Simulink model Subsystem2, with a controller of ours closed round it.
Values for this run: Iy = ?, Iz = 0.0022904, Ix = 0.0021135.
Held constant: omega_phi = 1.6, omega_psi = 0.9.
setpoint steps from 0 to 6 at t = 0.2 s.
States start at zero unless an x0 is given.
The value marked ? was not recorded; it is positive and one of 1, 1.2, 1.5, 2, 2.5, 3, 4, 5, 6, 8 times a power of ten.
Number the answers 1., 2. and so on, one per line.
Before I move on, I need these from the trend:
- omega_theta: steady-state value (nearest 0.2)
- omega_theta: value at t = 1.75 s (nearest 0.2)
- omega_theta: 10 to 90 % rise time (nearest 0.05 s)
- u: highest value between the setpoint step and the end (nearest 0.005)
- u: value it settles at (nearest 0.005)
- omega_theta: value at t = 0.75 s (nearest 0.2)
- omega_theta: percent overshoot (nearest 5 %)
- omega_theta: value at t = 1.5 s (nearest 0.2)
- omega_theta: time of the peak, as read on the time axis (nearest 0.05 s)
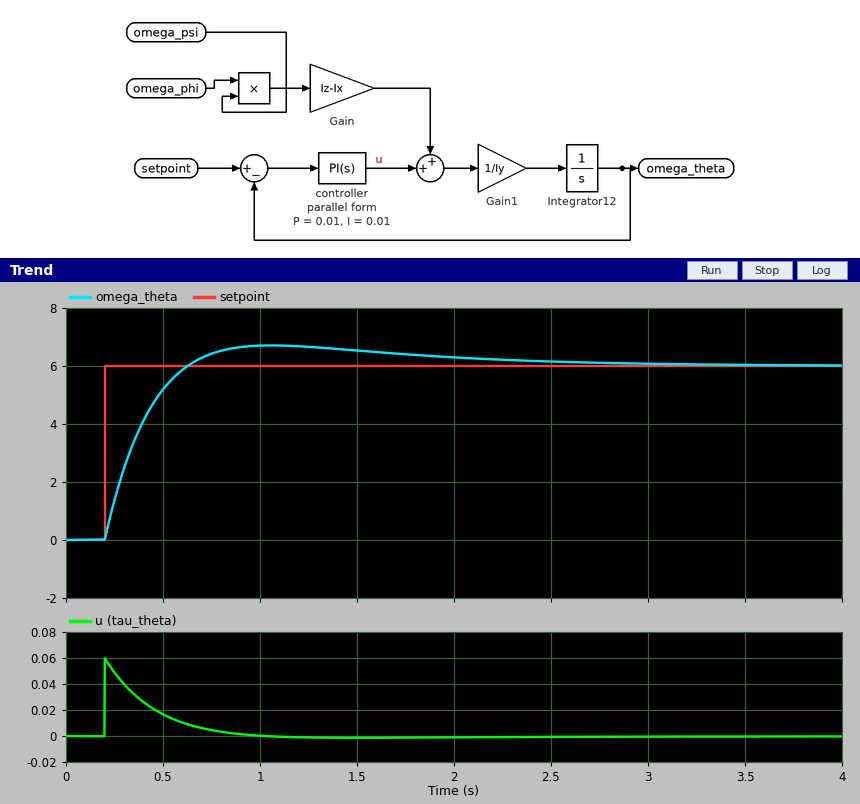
1. 6.0
2. 6.4
3. 0.30 s
4. 0.060
5. 0.000
6. 6.4
7. 10 %
8. 6.6
9. 1.05 s
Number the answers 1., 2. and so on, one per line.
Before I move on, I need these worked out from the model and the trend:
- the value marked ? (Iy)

1. 0.002
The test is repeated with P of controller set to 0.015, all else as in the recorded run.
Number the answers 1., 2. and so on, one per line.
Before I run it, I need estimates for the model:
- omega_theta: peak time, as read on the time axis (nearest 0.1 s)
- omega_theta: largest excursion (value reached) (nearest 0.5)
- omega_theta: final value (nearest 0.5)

1. 0.9 s
2. 6.5
3. 6.0
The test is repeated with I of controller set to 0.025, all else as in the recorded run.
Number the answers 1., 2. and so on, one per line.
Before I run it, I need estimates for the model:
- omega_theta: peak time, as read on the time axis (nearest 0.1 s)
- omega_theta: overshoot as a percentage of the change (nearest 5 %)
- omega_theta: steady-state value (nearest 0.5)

1. 0.8 s
2. 20 %
3. 6.0
